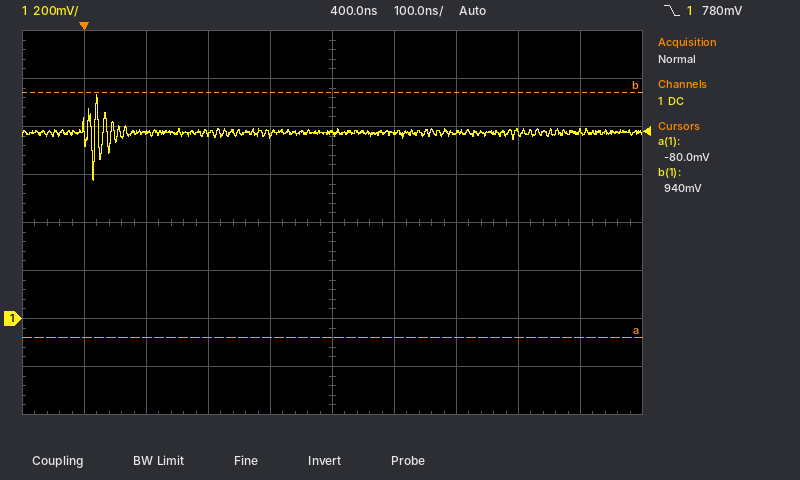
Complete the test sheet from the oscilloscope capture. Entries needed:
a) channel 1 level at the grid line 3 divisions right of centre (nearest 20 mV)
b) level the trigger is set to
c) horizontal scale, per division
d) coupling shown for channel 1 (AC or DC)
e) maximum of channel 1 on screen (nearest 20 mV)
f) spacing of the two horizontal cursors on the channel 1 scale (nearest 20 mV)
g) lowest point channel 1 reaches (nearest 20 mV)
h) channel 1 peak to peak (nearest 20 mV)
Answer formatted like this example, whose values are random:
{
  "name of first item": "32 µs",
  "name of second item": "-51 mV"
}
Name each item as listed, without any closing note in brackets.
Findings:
{
  "channel 1 level at the grid line 3 divisions right of centre": "780 mV",
  "level the trigger is set to": "780 mV",
  "horizontal scale, per division": "100 ns",
  "coupling shown for channel 1": "DC",
  "maximum of channel 1 on screen": "940 mV",
  "spacing of the two horizontal cursors on the channel 1 scale": "1.02 V",
  "lowest point channel 1 reaches": "580 mV",
  "channel 1 peak to peak": "360 mV"
}
